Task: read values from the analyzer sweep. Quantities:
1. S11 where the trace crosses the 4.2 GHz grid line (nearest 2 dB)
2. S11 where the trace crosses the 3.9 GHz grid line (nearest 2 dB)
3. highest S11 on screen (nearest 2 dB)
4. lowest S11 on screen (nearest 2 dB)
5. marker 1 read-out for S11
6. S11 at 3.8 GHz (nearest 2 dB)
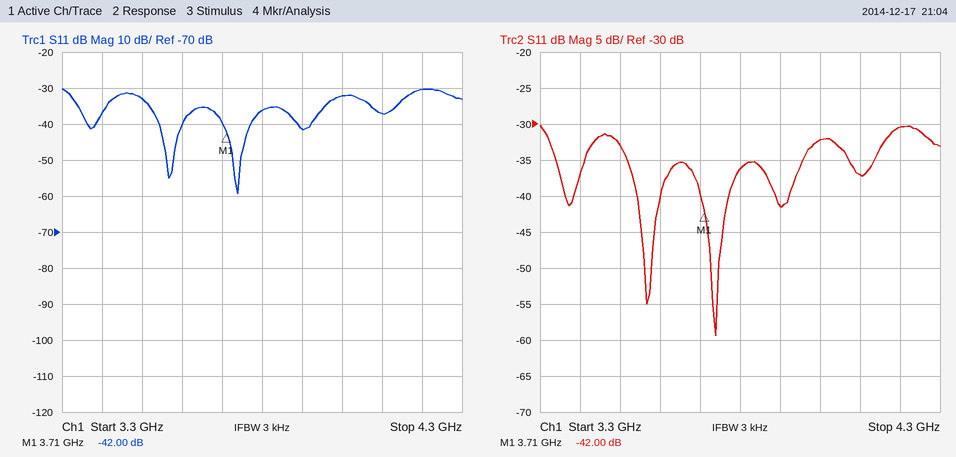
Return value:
-30 dB
-42 dB
-30 dB
-60 dB
-42.00 dB
-36 dB
